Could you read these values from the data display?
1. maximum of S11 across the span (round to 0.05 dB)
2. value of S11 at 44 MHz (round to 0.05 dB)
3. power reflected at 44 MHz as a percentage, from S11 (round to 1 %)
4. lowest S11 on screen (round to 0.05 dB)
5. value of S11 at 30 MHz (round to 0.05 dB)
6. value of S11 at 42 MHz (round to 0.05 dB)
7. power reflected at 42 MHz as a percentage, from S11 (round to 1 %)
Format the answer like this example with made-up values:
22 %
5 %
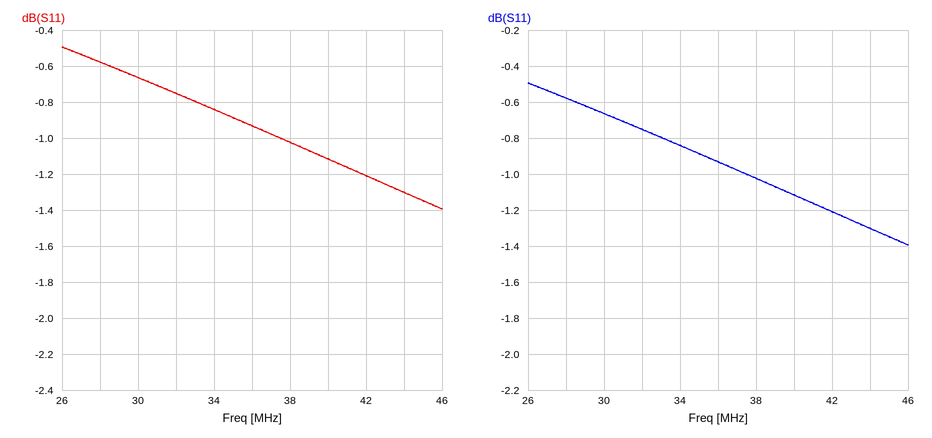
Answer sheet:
-0.50 dB
-1.30 dB
74 %
-1.40 dB
-0.65 dB
-1.20 dB
76 %
